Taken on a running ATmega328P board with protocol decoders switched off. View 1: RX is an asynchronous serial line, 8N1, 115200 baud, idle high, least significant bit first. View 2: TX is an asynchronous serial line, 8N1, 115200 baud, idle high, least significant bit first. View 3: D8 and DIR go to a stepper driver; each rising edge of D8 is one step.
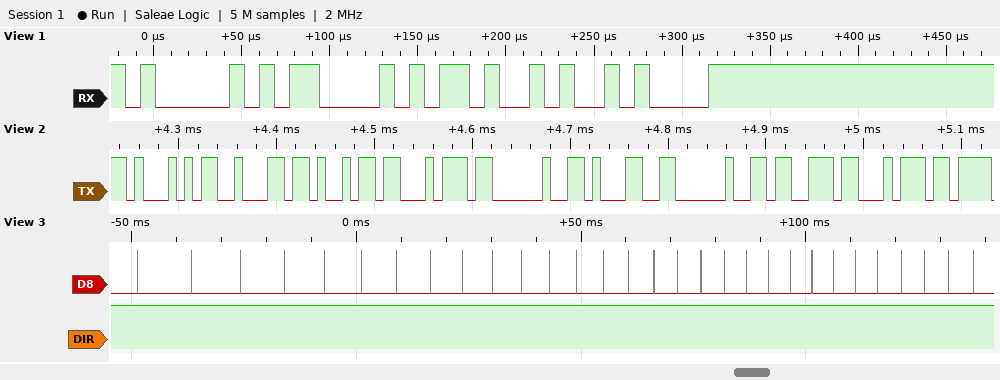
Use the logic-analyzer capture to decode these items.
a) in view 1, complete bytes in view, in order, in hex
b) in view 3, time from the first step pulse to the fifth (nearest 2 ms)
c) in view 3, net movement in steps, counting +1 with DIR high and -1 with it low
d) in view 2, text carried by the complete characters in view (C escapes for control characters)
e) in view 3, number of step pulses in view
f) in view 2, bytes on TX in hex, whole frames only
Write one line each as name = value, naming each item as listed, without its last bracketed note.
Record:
in view 1, complete bytes in view, in order, in hex = 41 43 4B 0A
in view 3, time from the first step pulse to the fifth = 42 ms
in view 3, net movement in steps, counting +1 with DIR high and -1 with it low = +30
in view 2, text carried by the complete characters in view = "Qbit 1 st"
in view 3, number of step pulses in view = 30
in view 2, bytes on TX in hex, whole frames only = 51 62 69 74 20 31 20 73 74
